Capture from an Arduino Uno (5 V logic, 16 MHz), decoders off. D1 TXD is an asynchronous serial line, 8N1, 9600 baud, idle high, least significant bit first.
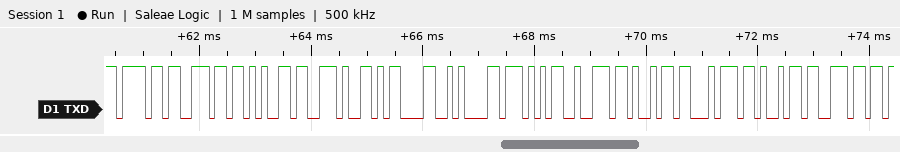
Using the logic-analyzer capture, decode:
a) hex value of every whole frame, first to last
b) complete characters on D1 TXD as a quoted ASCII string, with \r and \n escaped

6F 6E 65 2E 0D 0A 57 72 69 74 69 6E
"one.\r\nWritin"
